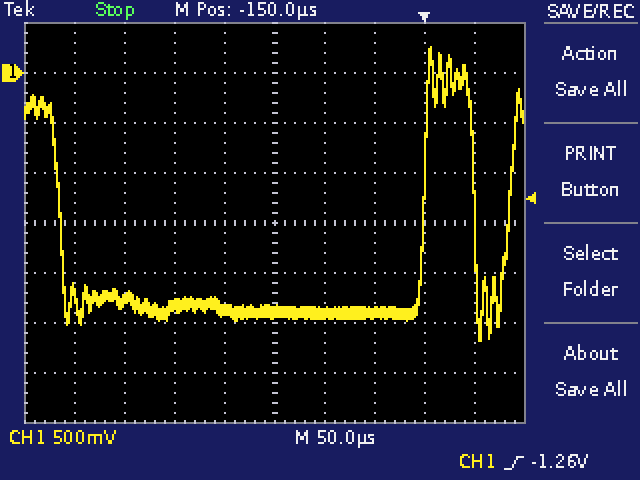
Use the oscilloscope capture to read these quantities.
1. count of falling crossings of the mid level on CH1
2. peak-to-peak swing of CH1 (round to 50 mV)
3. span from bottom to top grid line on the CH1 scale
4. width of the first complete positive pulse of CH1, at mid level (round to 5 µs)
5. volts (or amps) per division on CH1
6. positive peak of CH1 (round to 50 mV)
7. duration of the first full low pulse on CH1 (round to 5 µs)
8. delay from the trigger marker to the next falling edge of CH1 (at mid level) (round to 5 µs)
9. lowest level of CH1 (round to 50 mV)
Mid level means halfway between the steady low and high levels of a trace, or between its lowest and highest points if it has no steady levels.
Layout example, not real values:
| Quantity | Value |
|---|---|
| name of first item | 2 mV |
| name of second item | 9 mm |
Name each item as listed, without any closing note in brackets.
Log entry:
| Quantity | Value |
|---|---|
| count of falling crossings of the mid level on CH1 | 2 |
| peak-to-peak swing of CH1 | 2.95 V |
| span from bottom to top grid line on the CH1 scale | 4 V |
| width of the first complete positive pulse of CH1, at mid level | 50 µs |
| volts (or amps) per division on CH1 | 500 mV |
| positive peak of CH1 | 250 mV |
| duration of the first full low pulse on CH1 | 365 µs |
| delay from the trigger marker to the next falling edge of CH1 (at mid level) | 50 µs |
| lowest level of CH1 | -2.70 V |
